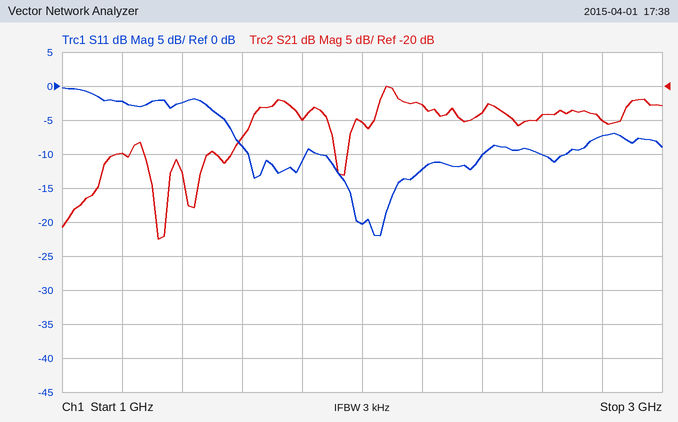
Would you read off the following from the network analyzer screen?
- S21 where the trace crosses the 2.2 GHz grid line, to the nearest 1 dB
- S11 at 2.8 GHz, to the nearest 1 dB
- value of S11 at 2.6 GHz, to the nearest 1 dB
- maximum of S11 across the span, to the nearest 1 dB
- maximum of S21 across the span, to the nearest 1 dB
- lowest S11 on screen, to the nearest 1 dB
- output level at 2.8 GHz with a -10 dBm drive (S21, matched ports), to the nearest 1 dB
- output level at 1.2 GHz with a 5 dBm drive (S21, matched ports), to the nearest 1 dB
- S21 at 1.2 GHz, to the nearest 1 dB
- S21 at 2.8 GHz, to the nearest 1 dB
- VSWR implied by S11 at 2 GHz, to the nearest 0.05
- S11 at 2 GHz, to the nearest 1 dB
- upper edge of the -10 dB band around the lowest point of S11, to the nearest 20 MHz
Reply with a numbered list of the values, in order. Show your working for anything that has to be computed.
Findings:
1. -23 dB
2. -7 dB
3. -10 dB
4. 0 dB
5. -20 dB
6. -22 dB
7. -10 dBm + (-25 dB) = -35 dBm
8. 5 dBm + (-30 dB) = -25 dBm
9. -30 dB
10. -25 dB
11. |Γ| = 10^(-20/20) = 0.1000; VSWR = (1 + 0.1000)/(1 − 0.1000) ≈ 1.22, so 1.20 to the nearest 0.05
12. -20 dB
13. 2.40 GHz
